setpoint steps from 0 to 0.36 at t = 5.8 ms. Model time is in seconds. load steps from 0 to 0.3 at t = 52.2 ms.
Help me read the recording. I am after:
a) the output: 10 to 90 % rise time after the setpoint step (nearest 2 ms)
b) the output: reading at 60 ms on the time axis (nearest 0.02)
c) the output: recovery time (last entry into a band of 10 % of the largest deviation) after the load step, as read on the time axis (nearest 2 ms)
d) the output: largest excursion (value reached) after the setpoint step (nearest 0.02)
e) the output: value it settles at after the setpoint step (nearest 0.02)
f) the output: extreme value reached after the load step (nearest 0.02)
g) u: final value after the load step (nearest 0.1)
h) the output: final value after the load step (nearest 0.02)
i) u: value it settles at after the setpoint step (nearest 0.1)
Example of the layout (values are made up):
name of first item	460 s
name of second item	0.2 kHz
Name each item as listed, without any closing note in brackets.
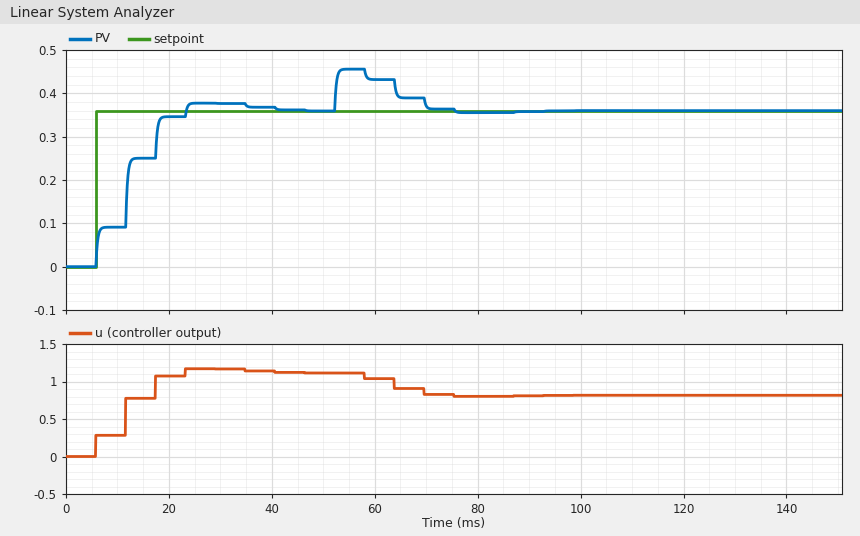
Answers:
the output: 10 to 90 % rise time after the setpoint step	12 ms
the output: reading at 60 ms on the time axis	0.44
the output: recovery time (last entry into a band of 10 % of the largest deviation) after the load step, as read on the time axis	70 ms
the output: largest excursion (value reached) after the setpoint step	0.38
the output: value it settles at after the setpoint step	0.36
the output: extreme value reached after the load step	0.46
u: final value after the load step	0.8
the output: final value after the load step	0.36
u: value it settles at after the setpoint step	1.1
